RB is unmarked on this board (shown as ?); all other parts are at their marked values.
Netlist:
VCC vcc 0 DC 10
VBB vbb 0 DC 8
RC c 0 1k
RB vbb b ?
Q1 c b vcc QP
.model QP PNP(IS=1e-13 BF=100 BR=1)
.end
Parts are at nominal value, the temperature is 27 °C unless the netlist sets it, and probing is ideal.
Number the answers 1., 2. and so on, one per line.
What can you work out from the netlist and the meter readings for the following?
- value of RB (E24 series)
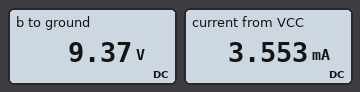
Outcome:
1. 39 kΩ
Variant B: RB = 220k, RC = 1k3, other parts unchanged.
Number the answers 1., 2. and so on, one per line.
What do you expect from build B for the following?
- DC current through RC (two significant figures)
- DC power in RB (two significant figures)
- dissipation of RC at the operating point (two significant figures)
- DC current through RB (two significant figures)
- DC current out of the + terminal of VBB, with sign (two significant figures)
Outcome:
1. 640 µA
2. 9.1 µW
3. 540 µW
4. 6.4 µA
5. -6.4 µA
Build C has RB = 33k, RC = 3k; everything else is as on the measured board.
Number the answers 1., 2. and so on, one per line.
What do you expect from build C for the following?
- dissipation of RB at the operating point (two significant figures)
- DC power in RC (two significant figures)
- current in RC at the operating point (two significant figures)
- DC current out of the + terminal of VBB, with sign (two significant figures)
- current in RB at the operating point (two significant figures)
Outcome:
1. 57 µW
2. 32 mW
3. 3.3 mA
4. -42 µA
5. 42 µA
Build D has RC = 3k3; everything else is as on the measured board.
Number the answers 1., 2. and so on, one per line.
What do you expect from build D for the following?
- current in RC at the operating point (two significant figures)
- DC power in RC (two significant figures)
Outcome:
1. 3.0 mA
2. 29 mW
